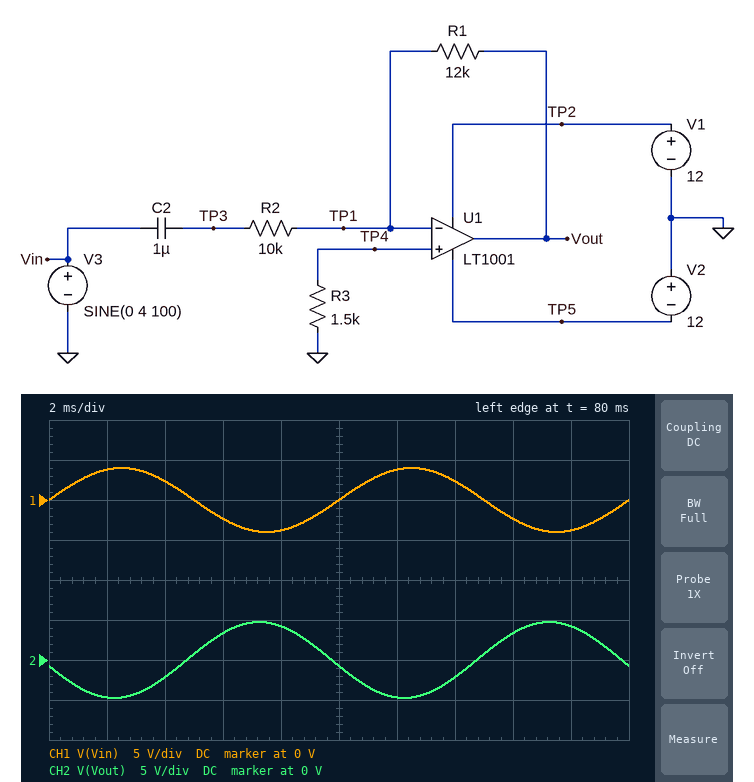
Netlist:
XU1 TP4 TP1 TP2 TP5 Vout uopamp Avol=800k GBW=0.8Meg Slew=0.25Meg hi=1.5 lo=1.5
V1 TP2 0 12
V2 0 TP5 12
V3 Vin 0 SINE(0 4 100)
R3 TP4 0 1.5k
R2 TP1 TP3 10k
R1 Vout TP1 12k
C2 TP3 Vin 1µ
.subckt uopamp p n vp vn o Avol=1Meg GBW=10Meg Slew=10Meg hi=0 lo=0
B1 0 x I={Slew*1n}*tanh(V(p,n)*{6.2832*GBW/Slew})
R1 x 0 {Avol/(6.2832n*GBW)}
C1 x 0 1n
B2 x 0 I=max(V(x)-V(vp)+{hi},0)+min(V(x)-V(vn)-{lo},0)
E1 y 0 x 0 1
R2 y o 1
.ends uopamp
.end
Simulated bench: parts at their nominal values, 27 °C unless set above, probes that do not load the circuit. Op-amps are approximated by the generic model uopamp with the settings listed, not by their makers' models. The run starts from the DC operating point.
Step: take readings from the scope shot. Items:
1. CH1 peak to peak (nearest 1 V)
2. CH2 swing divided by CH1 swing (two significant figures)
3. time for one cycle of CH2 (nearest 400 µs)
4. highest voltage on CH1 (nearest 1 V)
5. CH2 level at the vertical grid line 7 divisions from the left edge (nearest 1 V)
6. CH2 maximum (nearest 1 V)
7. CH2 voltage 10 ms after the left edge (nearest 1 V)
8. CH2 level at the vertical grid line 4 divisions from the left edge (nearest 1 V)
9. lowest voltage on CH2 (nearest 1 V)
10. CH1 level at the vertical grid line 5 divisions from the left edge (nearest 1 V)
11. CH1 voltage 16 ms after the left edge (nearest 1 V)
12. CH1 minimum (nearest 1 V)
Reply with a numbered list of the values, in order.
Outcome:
1. 8 V
2. 1.2
3. 10.0 ms
4. 4 V
5. -2 V
6. 5 V
7. -1 V
8. 4 V
9. -5 V
10. 0 V
11. -2 V
12. -4 V
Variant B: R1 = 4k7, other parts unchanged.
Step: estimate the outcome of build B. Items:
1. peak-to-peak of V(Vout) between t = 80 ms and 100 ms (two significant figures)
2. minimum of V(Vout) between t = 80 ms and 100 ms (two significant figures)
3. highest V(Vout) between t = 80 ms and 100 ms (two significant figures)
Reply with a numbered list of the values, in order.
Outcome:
1. 3.7 V
2. -1.9 V
3. 1.9 V
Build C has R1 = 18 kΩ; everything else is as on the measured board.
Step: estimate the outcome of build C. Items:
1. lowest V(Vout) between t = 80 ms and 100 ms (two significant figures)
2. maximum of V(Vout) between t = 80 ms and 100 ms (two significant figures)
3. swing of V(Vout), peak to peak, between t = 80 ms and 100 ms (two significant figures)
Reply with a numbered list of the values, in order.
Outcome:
1. -7.1 V
2. 7.1 V
3. 14 V
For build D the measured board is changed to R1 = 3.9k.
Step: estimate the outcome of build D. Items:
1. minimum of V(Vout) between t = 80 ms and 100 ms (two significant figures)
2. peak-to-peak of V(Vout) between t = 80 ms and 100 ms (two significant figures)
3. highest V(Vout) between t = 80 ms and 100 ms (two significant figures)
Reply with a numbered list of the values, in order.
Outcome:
1. -1.5 V
2. 3.1 V
3. 1.5 V
